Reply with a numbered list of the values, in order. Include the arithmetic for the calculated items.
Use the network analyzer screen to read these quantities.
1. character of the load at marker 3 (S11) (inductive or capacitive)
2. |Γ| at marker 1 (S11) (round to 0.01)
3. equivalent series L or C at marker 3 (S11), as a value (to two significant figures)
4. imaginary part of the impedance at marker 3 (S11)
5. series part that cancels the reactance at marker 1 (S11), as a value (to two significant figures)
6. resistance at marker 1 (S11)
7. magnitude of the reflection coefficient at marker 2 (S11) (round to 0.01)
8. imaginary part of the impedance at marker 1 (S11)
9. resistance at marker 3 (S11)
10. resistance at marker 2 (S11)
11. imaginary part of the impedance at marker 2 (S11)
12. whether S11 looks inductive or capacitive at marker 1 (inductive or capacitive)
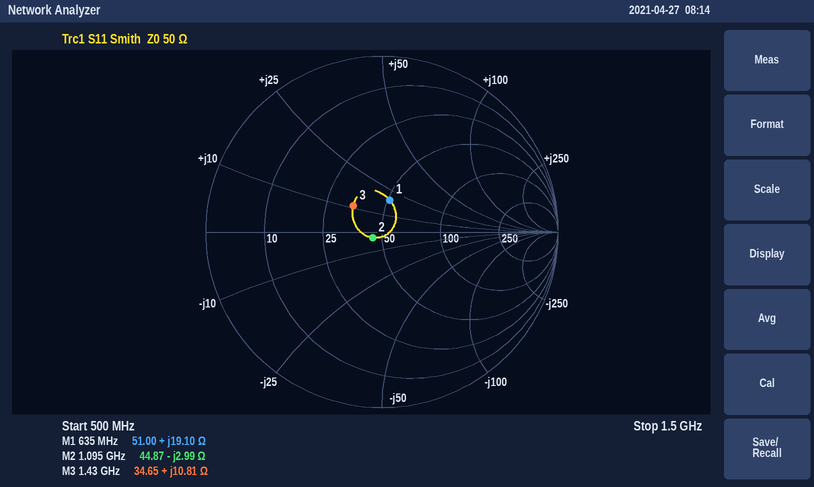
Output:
1. inductive
2. 0.19
3. L = 10.81 Ω/(2π × 1.43 GHz) ≈ 1.2 nH
4. +10.81 Ω
5. C = 1/(2π × 635 MHz × 19.1 Ω) ≈ 13 pF
6. 51.00 Ω
7. 0.06
8. +19.10 Ω
9. 34.65 Ω
10. 44.87 Ω
11. -2.99 Ω
12. inductive
